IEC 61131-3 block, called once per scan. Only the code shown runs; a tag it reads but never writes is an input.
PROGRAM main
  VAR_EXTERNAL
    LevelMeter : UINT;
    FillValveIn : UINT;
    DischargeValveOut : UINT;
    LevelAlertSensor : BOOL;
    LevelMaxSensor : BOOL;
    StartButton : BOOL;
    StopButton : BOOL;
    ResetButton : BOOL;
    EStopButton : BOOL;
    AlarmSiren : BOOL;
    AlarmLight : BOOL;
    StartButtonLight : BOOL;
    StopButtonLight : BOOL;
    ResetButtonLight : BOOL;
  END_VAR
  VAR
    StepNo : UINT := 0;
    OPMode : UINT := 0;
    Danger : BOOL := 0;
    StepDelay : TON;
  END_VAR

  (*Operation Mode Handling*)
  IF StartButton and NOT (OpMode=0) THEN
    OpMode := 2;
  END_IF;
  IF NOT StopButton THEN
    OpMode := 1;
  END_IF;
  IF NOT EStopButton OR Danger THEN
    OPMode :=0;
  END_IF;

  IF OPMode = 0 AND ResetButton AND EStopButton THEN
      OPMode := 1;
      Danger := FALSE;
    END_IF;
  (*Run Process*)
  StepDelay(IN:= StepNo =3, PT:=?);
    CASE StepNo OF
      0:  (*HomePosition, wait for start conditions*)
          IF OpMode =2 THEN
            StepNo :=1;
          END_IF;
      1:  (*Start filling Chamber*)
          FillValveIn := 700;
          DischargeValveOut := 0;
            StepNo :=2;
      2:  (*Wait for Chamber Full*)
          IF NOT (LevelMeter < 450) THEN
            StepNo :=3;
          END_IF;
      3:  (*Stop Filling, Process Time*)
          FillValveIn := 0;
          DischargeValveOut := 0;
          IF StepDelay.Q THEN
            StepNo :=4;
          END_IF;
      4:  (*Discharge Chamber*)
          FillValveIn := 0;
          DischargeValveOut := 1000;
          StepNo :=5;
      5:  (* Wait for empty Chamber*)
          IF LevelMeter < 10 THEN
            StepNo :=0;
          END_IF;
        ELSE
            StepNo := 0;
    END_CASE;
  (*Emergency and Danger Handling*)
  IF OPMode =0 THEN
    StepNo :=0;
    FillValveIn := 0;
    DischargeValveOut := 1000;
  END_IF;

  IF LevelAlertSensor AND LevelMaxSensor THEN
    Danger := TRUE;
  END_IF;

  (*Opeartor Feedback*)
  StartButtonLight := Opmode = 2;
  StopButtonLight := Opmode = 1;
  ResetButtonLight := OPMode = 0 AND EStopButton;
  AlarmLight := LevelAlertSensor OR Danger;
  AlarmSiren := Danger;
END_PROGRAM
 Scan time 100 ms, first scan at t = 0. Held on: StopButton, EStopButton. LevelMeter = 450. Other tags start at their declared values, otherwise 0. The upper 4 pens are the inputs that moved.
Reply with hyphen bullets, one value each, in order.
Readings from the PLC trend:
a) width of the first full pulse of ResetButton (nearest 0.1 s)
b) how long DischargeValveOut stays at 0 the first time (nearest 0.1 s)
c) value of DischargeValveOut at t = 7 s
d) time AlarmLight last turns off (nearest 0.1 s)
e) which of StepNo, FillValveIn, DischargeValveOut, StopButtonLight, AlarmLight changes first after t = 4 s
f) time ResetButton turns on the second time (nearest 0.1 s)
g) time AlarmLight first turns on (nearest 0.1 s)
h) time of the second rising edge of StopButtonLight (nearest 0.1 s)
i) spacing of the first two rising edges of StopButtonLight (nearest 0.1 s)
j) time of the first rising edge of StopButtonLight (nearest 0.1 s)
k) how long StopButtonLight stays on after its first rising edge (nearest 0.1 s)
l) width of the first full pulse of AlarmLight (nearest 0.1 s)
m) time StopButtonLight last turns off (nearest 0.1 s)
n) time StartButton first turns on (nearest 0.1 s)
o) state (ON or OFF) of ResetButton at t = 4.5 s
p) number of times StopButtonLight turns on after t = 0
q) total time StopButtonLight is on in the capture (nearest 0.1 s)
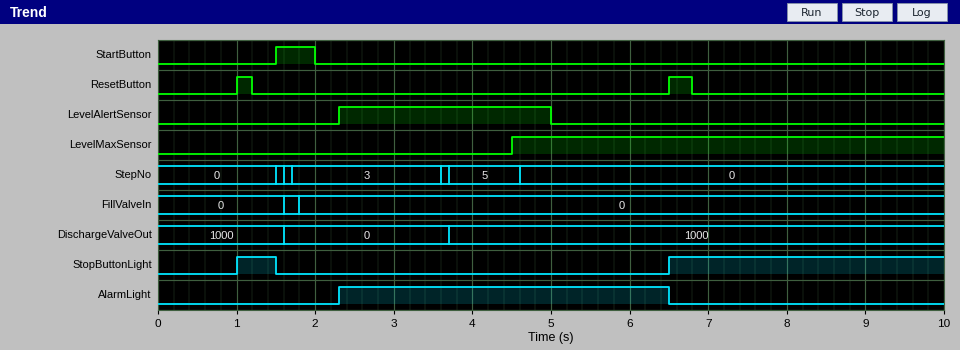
- 0.2 s
- 2.1 s
- 1000
- 6.5 s
- StepNo
- 6.5 s
- 2.3 s
- 6.5 s
- 5.5 s
- 1.0 s
- 0.5 s
- 4.2 s
- 1.5 s
- 1.5 s
- OFF
- 2
- 4.0 s
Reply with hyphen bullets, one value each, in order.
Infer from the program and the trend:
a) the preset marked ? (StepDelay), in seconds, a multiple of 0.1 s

- 1.8 s
